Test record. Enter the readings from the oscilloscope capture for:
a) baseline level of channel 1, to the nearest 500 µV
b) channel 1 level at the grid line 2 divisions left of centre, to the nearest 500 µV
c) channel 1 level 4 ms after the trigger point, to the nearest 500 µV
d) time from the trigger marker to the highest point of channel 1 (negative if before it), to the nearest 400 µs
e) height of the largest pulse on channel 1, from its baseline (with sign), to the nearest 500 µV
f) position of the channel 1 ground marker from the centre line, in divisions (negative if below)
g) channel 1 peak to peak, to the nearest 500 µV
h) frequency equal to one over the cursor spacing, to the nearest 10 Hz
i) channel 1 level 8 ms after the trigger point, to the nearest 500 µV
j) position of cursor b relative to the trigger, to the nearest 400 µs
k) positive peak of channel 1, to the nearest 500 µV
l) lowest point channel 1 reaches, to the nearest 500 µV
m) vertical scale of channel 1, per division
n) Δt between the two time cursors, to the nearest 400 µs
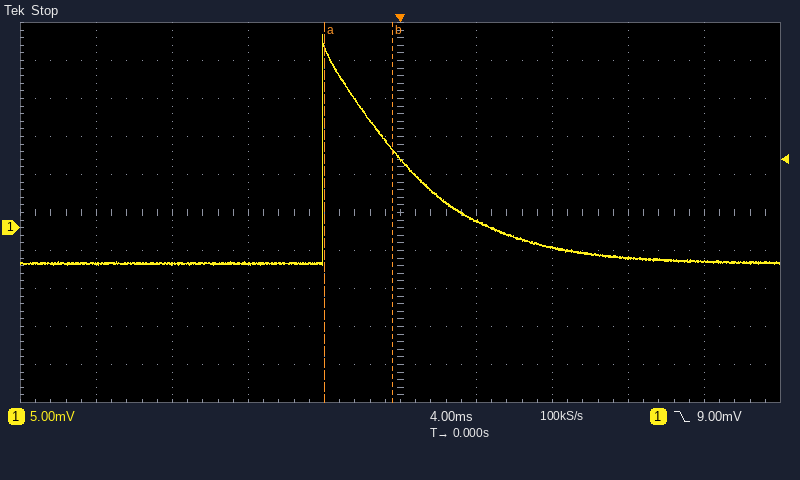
-4.5 mV
-4.5 mV
1.0 mV
-4.0 ms
+30.0 mV
-0.4 div
30.5 mV
280 Hz
-2.5 mV
-400 µs
25.5 mV
-5.0 mV
5 mV
3.6 ms
